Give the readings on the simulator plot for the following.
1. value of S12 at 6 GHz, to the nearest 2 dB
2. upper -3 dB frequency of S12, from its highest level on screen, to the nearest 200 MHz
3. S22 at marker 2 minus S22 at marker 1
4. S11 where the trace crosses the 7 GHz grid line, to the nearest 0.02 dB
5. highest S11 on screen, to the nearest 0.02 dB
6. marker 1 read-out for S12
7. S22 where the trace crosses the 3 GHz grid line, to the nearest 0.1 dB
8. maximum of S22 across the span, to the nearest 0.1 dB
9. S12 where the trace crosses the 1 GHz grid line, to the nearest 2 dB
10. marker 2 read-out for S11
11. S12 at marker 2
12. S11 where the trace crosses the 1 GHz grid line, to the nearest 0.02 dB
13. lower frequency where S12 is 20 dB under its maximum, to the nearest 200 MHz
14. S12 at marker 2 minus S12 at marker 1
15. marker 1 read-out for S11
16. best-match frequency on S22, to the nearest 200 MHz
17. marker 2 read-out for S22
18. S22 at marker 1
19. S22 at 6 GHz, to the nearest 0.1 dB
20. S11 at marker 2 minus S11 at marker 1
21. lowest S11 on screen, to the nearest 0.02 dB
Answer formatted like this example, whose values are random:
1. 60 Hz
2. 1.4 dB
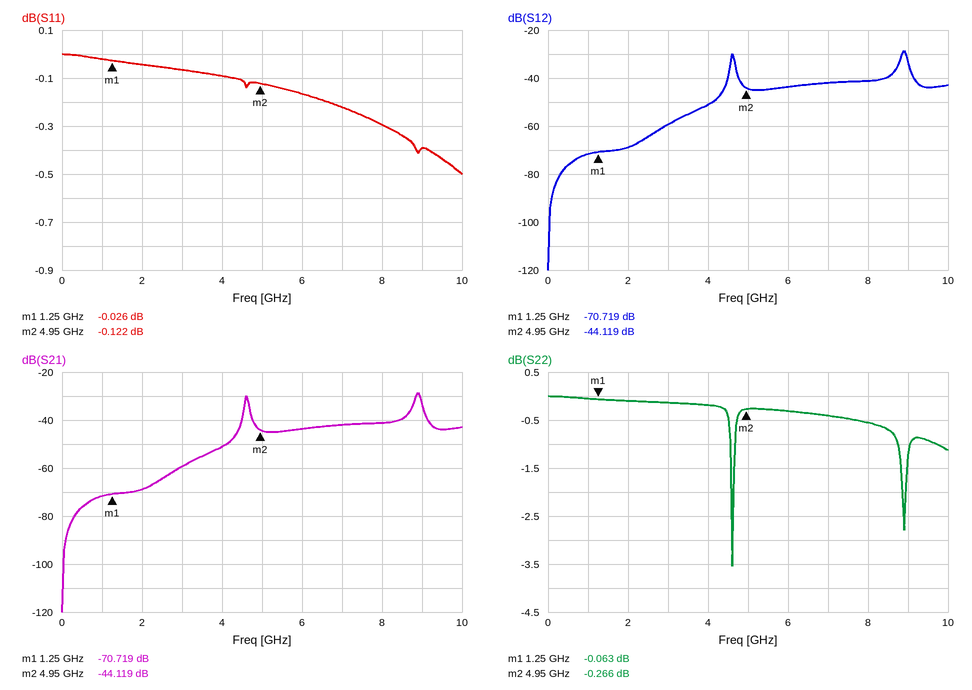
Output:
1. -44 dB
2. 9.0 GHz
3. -0.203 dB
4. -0.22 dB
5. 0.00 dB
6. -70.719 dB
7. -0.1 dB
8. 0.0 dB
9. -72 dB
10. -0.122 dB
11. -44.119 dB
12. -0.02 dB
13. 4.2 GHz
14. 26.600 dB
15. -0.026 dB
16. 4.6 GHz
17. -0.266 dB
18. -0.063 dB
19. -0.3 dB
20. -0.096 dB
21. -0.50 dB
